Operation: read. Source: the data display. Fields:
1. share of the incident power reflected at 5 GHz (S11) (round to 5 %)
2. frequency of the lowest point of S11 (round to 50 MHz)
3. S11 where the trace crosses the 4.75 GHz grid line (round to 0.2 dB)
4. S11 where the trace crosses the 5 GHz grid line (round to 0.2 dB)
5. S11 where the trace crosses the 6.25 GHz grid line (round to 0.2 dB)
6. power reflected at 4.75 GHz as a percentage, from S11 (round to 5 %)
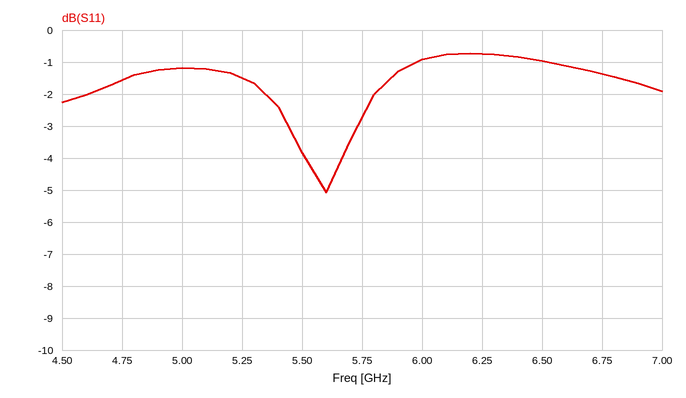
75 %
5.60 GHz
-1.6 dB
-1.2 dB
-0.8 dB
70 %
